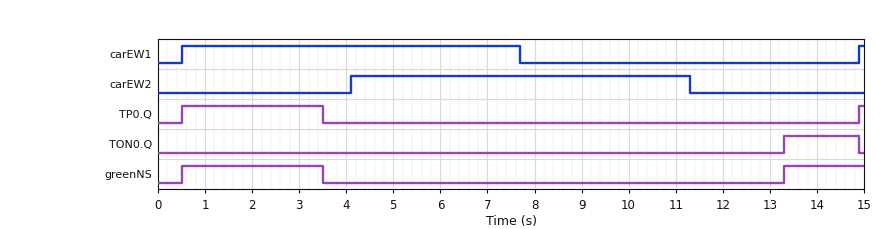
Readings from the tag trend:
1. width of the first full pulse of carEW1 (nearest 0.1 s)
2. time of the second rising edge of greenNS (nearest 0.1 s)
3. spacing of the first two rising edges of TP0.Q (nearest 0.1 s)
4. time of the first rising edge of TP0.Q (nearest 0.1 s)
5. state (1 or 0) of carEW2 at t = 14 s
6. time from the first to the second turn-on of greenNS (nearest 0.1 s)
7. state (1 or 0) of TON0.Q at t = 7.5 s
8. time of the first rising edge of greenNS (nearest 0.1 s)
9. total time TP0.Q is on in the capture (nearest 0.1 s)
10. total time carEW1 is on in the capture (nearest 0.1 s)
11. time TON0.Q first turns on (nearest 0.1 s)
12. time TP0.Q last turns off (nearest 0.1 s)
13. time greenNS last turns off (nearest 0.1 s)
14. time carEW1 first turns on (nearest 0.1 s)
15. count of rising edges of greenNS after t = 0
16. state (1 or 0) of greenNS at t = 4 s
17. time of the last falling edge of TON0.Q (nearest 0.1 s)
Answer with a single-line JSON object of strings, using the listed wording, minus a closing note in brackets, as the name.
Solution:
{"width of the first full pulse of carEW1": "7.2 s", "time of the second rising edge of greenNS": "13.3 s", "spacing of the first two rising edges of TP0.Q": "14.4 s", "time of the first rising edge of TP0.Q": "0.5 s", "state (1 or 0) of carEW2 at t = 14 s": "0", "time from the first to the second turn-on of greenNS": "12.8 s", "state (1 or 0) of TON0.Q at t = 7.5 s": "0", "time of the first rising edge of greenNS": "0.5 s", "total time TP0.Q is on in the capture": "3.1 s", "total time carEW1 is on in the capture": "7.3 s", "time TON0.Q first turns on": "13.3 s", "time TP0.Q last turns off": "3.5 s", "time greenNS last turns off": "3.5 s", "time carEW1 first turns on": "0.5 s", "count of rising edges of greenNS after t = 0": "2", "state (1 or 0) of greenNS at t = 4 s": "0", "time of the last falling edge of TON0.Q": "14.9 s"}
